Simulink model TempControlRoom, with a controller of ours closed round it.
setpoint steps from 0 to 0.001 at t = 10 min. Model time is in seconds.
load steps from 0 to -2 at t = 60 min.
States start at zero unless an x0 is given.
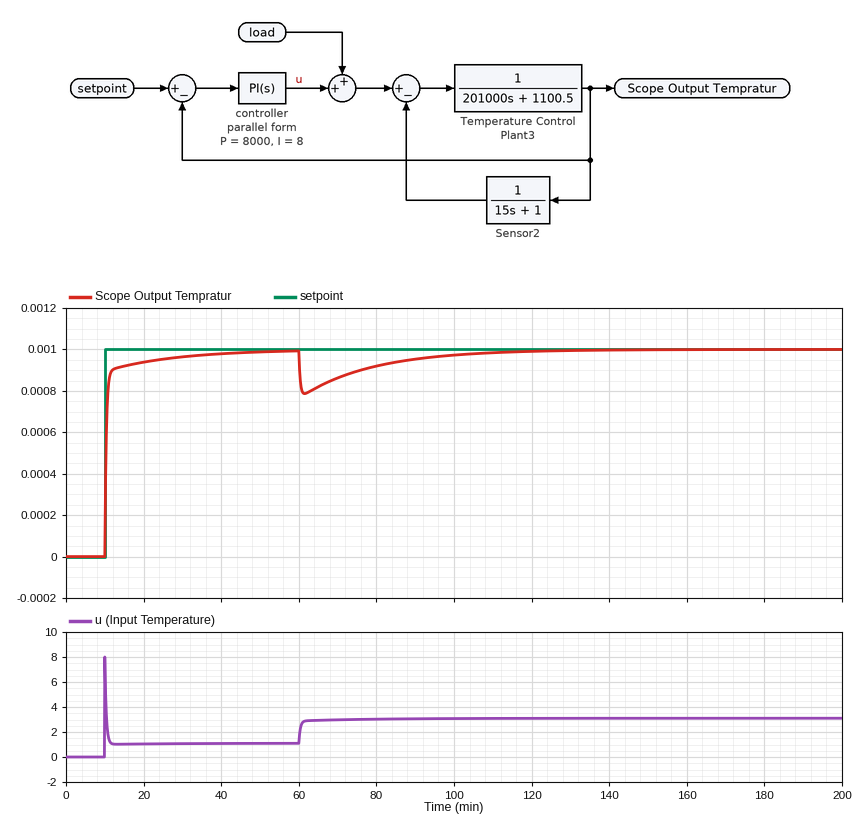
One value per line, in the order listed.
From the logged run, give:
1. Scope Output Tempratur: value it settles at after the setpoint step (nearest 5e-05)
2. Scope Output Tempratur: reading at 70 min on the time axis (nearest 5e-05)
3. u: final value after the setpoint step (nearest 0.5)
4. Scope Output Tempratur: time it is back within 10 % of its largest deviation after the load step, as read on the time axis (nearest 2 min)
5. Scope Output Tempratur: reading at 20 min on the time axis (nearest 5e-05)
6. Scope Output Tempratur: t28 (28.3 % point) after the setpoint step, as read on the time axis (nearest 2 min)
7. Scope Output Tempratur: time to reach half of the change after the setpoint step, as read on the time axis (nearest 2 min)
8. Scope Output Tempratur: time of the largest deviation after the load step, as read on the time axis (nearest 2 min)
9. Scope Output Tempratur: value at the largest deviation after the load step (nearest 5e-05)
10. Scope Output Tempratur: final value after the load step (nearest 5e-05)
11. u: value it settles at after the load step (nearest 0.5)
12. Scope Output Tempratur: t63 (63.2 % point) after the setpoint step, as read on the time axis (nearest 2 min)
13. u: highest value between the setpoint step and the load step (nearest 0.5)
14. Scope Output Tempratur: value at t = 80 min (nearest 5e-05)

0.00100
0.00085
1.0
106 min
0.00095
10 min
10 min
62 min
0.00080
0.00100
3.0
10 min
8.0
0.00090
